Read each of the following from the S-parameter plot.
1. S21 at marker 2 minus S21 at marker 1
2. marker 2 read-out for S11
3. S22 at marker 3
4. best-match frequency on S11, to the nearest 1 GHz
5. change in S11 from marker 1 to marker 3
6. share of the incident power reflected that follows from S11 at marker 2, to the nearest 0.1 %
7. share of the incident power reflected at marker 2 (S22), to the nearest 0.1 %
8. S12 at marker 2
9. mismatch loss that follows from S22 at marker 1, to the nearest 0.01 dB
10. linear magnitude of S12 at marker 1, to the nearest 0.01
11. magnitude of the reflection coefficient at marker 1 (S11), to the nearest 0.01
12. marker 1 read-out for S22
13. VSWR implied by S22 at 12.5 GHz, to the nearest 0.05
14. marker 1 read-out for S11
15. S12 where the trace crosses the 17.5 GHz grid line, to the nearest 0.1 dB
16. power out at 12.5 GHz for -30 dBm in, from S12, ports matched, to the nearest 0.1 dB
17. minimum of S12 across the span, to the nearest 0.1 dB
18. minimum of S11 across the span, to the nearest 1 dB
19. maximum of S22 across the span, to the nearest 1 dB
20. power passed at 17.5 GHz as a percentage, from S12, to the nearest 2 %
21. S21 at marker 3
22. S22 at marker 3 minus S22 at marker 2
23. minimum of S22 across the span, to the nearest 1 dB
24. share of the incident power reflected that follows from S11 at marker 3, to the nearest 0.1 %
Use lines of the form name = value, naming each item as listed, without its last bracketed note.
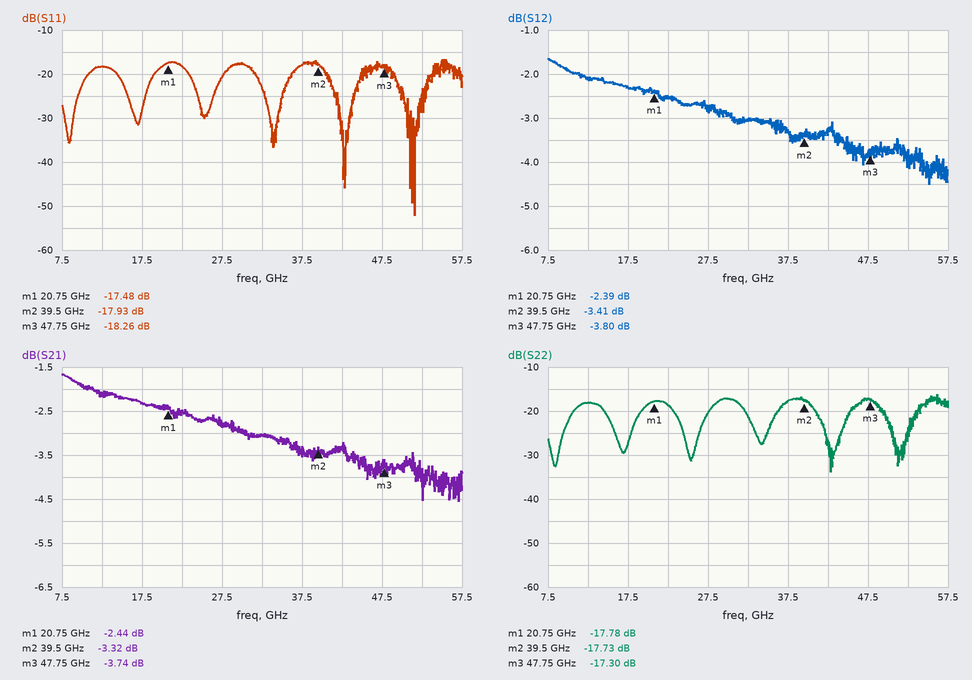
S21 at marker 2 minus S21 at marker 1 = -0.88 dB
marker 2 read-out for S11 = -17.93 dB
S22 at marker 3 = -17.30 dB
best-match frequency on S11, to the nearest 1 GHz = 52 GHz
change in S11 from marker 1 to marker 3 = -0.78 dB
share of the incident power reflected that follows from S11 at marker 2, to the nearest 0.1 % = 1.6 %
share of the incident power reflected at marker 2 (S22), to the nearest 0.1 % = 1.7 %
S12 at marker 2 = -3.41 dB
mismatch loss that follows from S22 at marker 1, to the nearest 0.01 dB = 0.07 dB
linear magnitude of S12 at marker 1, to the nearest 0.01 = 0.76
magnitude of the reflection coefficient at marker 1 (S11), to the nearest 0.01 = 0.13
marker 1 read-out for S22 = -17.78 dB
VSWR implied by S22 at 12.5 GHz, to the nearest 0.05 = 1.30
marker 1 read-out for S11 = -17.48 dB
S12 where the trace crosses the 17.5 GHz grid line, to the nearest 0.1 dB = -2.3 dB
power out at 12.5 GHz for -30 dBm in, from S12, ports matched, to the nearest 0.1 dB = -32.1 dBm
minimum of S12 across the span, to the nearest 0.1 dB = -4.5 dB
minimum of S11 across the span, to the nearest 1 dB = -52 dB
maximum of S22 across the span, to the nearest 1 dB = -16 dB
power passed at 17.5 GHz as a percentage, from S12, to the nearest 2 % = 58 %
S21 at marker 3 = -3.74 dB
S22 at marker 3 minus S22 at marker 2 = 0.43 dB
minimum of S22 across the span, to the nearest 1 dB = -34 dB
share of the incident power reflected that follows from S11 at marker 3, to the nearest 0.1 % = 1.5 %
